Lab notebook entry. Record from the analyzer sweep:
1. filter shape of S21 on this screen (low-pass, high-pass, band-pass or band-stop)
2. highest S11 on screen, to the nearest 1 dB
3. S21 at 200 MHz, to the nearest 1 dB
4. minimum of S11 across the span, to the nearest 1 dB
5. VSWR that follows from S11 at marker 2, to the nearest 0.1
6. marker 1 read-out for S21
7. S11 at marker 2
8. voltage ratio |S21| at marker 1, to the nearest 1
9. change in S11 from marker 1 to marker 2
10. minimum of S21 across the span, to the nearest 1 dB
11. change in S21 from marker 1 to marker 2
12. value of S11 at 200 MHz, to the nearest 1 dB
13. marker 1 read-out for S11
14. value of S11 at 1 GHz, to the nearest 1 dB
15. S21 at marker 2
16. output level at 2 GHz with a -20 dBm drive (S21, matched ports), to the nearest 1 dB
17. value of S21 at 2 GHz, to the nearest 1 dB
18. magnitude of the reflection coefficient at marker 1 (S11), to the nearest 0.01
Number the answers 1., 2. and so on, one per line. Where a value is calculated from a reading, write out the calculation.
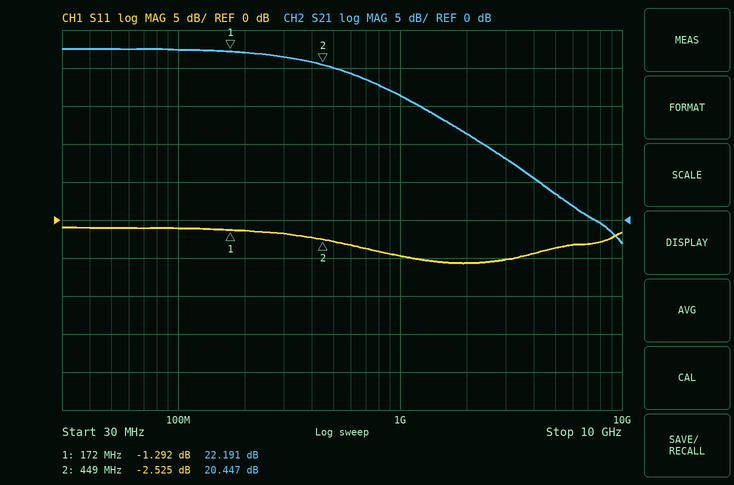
1. low-pass
2. -1 dB
3. 22 dB
4. -6 dB
5. (1 + 0.7477)/(1 − 0.7477) ≈ 6.9
6. 22.191 dB
7. -2.525 dB
8. 10^(22.191/20) ≈ 13
9. -2.525 − (-1.292) = -1.233 dB
10. -3 dB
11. 20.447 − (22.191) = -1.744 dB
12. -1 dB
13. -1.292 dB
14. -5 dB
15. 20.447 dB
16. -20 dBm + (11 dB) = -9 dBm
17. 11 dB
18. 10^(-1.292/20) ≈ 0.86
